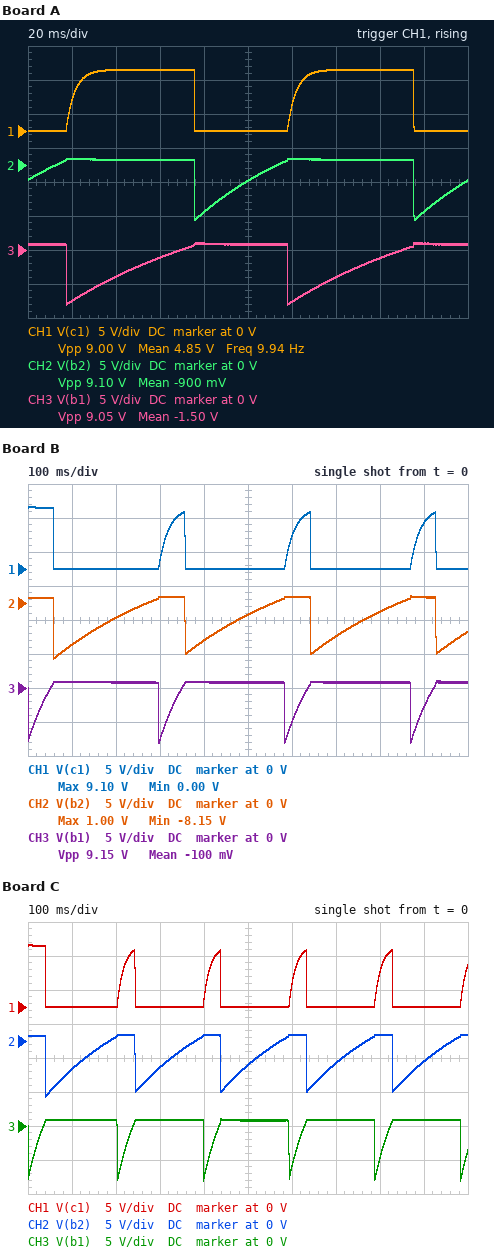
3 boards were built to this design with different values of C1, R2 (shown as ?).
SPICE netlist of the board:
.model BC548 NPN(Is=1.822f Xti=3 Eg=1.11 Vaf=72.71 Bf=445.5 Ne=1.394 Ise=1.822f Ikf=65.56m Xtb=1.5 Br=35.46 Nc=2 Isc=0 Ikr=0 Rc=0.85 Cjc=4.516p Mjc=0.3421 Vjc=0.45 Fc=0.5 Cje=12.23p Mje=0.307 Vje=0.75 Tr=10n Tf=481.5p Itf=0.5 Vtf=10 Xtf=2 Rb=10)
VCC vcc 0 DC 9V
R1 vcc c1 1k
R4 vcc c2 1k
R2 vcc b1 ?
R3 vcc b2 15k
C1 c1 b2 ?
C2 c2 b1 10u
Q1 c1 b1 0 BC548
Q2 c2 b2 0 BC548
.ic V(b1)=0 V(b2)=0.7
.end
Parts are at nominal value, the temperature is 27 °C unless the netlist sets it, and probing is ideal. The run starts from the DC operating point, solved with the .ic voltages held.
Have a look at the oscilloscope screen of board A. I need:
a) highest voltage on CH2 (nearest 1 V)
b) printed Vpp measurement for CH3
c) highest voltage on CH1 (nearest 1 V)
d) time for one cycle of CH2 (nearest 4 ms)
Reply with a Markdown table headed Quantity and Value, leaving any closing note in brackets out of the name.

| Quantity | Value |
|---|---|
| highest voltage on CH2 | 1 V |
| printed Vpp measurement for CH3 | 9.05 V |
| highest voltage on CH1 | 9 V |
| time for one cycle of CH2 | 100 ms |
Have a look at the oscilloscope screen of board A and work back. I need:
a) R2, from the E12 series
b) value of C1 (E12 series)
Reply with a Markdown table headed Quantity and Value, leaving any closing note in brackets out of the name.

| Quantity | Value |
|---|---|
| R2, from the E12 series | 8.2 kΩ |
| value of C1 | 3.9 µF |
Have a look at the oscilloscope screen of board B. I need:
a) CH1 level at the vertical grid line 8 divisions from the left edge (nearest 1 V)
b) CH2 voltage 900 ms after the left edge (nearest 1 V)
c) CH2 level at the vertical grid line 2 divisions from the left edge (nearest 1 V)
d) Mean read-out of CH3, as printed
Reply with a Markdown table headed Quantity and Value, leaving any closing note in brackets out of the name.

| Quantity | Value |
|---|---|
| CH1 level at the vertical grid line 8 divisions from the left edge | 0 V |
| CH2 voltage 900 ms after the left edge | 1 V |
| CH2 level at the vertical grid line 2 divisions from the left edge | -2 V |
| Mean read-out of CH3, as printed | -100 mV |
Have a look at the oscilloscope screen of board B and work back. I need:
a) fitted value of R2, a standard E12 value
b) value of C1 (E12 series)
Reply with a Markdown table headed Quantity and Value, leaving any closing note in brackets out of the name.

| Quantity | Value |
|---|---|
| fitted value of R2, a standard E12 value | 8.2 kΩ |
| value of C1 | 22 µF |
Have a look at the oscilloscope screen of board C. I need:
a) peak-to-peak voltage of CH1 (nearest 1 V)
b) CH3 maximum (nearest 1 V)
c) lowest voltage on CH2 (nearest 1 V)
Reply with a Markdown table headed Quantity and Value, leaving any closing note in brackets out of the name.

| Quantity | Value |
|---|---|
| peak-to-peak voltage of CH1 | 9 V |
| CH3 maximum | 1 V |
| lowest voltage on CH2 | -8 V |
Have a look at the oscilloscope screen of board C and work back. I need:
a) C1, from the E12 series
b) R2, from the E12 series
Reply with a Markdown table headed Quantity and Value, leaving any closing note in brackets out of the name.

| Quantity | Value |
|---|---|
| C1, from the E12 series | 15 µF |
| R2, from the E12 series | 5.6 kΩ |
